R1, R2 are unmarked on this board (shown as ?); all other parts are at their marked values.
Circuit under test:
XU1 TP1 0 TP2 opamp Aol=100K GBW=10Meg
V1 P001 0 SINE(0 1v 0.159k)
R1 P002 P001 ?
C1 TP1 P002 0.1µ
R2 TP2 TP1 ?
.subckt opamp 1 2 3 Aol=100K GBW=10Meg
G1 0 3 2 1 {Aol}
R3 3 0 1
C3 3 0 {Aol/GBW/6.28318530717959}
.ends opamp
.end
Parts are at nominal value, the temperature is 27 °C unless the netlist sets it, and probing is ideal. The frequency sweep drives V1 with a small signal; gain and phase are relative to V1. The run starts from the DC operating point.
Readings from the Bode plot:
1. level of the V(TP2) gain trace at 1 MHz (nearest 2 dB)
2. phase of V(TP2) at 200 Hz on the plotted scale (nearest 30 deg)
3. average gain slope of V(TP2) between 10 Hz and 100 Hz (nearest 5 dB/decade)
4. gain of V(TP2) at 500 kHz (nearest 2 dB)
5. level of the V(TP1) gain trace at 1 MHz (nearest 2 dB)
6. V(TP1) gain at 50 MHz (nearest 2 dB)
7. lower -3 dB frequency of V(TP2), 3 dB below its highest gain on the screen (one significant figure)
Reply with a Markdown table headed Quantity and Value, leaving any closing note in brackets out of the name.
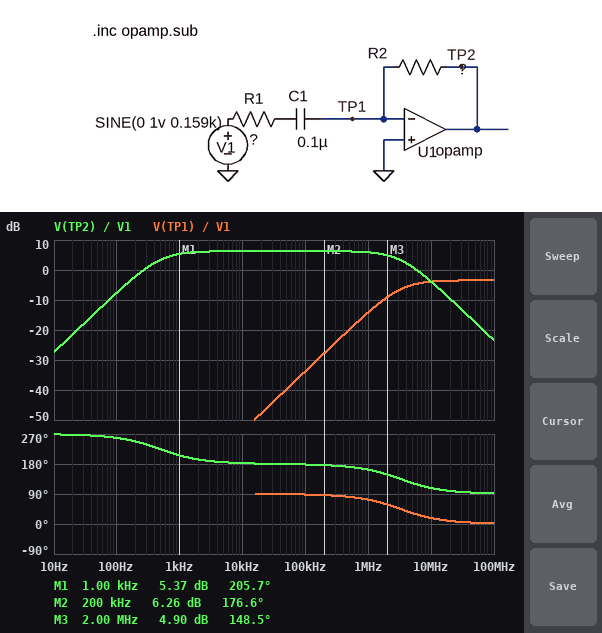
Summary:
| Quantity | Value |
|---|---|
| level of the V(TP2) gain trace at 1 MHz | 6 dB |
| phase of V(TP2) at 200 Hz on the plotted scale | 240 deg |
| average gain slope of V(TP2) between 10 Hz and 100 Hz | 20 dB/decade |
| gain of V(TP2) at 500 kHz | 6 dB |
| level of the V(TP1) gain trace at 1 MHz | -14 dB |
| V(TP1) gain at 50 MHz | -4 dB |
| lower -3 dB frequency of V(TP2), 3 dB below its highest gain on the screen | 500 Hz |
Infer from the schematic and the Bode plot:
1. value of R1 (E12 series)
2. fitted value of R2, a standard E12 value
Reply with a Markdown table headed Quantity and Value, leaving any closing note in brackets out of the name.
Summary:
| Quantity | Value |
|---|---|
| value of R1 | 3.3 kΩ |
| fitted value of R2, a standard E12 value | 6.8 kΩ |
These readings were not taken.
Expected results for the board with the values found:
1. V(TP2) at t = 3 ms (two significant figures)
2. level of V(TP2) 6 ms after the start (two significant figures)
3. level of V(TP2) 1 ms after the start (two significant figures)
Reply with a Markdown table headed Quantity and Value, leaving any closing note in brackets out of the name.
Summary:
| Quantity | Value |
|---|---|
| V(TP2) at t = 3 ms | 580 mV |
| level of V(TP2) 6 ms after the start | -530 mV |
| level of V(TP2) 1 ms after the start | -470 mV |
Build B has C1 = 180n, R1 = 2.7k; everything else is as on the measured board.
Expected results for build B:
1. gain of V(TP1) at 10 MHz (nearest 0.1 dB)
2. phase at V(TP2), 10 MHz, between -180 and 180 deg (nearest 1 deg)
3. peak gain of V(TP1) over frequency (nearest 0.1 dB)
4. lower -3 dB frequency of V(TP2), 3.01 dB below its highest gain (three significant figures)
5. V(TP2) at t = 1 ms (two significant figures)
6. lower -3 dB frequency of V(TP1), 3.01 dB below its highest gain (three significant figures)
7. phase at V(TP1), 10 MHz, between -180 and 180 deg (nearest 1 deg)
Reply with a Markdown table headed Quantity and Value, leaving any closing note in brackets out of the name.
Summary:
| Quantity | Value |
|---|---|
| gain of V(TP1) at 10 MHz | -3.2 dB |
| phase at V(TP2), 10 MHz, between -180 and 180 deg | 106 deg |
| peak gain of V(TP1) over frequency | -2.9 dB |
| lower -3 dB frequency of V(TP2), 3.01 dB below its highest gain | 327 Hz |
| V(TP2) at t = 1 ms | -810 mV |
| lower -3 dB frequency of V(TP1), 3.01 dB below its highest gain | 2.84 MHz |
| phase at V(TP1), 10 MHz, between -180 and 180 deg | 16 deg |
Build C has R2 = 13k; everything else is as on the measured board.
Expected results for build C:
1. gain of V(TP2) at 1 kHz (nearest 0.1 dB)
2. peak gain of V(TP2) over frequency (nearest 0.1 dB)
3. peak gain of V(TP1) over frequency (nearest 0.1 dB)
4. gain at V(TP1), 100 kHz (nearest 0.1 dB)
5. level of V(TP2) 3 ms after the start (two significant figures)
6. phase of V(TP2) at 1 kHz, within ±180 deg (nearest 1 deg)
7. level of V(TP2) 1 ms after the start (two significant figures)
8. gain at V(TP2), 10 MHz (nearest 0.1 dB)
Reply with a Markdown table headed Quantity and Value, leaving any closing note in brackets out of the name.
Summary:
| Quantity | Value |
|---|---|
| gain of V(TP2) at 1 kHz | 11.0 dB |
| peak gain of V(TP2) over frequency | 11.9 dB |
| peak gain of V(TP1) over frequency | -2.0 dB |
| gain at V(TP1), 100 kHz | -28.1 dB |
| level of V(TP2) 3 ms after the start | 1.1 V |
| phase of V(TP2) at 1 kHz, within ±180 deg | -154 deg |
| level of V(TP2) 1 ms after the start | -900 mV |
| gain at V(TP2), 10 MHz | -2.1 dB |
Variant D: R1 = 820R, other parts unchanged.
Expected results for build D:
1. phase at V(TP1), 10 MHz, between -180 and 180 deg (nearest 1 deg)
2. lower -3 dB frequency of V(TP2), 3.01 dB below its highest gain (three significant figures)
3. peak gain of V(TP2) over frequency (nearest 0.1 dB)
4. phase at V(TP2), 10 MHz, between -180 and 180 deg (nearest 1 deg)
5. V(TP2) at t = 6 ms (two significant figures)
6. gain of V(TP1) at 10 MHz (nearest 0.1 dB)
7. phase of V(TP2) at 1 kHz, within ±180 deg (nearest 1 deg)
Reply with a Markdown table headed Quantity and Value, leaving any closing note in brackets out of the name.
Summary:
| Quantity | Value |
|---|---|
| phase at V(TP1), 10 MHz, between -180 and 180 deg | 6 deg |
| lower -3 dB frequency of V(TP2), 3.01 dB below its highest gain | 1.94 kHz |
| peak gain of V(TP2) over frequency | 18.4 dB |
| phase at V(TP2), 10 MHz, between -180 and 180 deg | 96 deg |
| V(TP2) at t = 6 ms | -630 mV |
| gain of V(TP1) at 10 MHz | -1.0 dB |
| phase of V(TP2) at 1 kHz, within ±180 deg | -117 deg |
